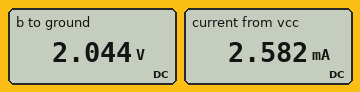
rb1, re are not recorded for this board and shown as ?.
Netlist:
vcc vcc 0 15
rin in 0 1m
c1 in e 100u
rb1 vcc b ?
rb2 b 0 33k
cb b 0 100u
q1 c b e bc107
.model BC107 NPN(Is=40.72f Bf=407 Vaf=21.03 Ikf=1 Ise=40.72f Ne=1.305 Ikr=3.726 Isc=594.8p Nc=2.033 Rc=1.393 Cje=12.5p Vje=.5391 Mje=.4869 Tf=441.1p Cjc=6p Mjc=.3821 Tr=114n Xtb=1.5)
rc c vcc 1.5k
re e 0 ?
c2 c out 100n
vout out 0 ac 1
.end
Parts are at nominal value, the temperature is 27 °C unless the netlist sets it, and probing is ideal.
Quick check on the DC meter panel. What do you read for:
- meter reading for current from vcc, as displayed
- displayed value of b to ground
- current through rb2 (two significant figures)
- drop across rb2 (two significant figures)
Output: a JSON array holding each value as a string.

["2.582 mA", "2.044 V", "62 µA", "2.0 V"]
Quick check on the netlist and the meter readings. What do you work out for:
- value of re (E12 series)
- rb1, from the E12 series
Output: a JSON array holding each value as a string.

["560 Ω", "180 kΩ"]
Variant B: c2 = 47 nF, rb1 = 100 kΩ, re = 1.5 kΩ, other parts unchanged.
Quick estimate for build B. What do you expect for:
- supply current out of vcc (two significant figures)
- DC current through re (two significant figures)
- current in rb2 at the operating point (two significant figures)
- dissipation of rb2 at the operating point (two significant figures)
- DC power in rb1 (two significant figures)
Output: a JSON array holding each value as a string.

["2.0 mA", "1.9 mA", "110 µA", "380 µW", "1.3 mW"]
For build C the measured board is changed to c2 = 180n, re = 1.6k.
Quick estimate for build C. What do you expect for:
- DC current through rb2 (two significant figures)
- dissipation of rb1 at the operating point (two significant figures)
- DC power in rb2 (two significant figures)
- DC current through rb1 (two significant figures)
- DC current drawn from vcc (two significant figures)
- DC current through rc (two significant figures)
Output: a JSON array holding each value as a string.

["67 µA", "910 µW", "150 µW", "71 µA", "1.1 mA", "990 µA"]
